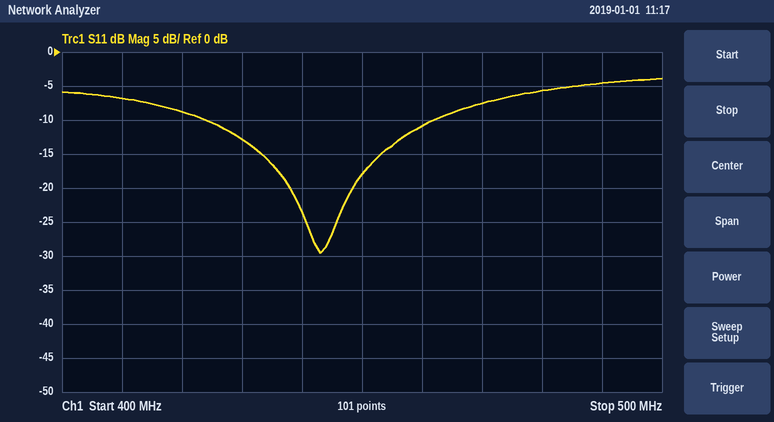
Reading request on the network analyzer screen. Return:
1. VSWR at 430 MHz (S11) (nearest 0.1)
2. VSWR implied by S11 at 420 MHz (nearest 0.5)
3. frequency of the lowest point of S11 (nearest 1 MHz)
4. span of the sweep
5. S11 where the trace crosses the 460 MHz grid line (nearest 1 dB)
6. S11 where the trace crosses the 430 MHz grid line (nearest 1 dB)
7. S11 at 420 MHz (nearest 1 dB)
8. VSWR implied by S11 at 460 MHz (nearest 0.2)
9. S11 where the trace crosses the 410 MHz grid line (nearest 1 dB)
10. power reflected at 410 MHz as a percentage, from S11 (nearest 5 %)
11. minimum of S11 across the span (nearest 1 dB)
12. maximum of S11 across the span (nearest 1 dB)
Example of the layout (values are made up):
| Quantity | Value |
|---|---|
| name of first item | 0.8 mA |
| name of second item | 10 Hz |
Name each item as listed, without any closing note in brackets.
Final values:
| Quantity | Value |
|---|---|
| VSWR at 430 MHz (S11) | 1.6 |
| VSWR implied by S11 at 420 MHz | 2.0 |
| frequency of the lowest point of S11 | 443 MHz |
| span of the sweep | 100 MHz |
| S11 where the trace crosses the 460 MHz grid line | -11 dB |
| S11 where the trace crosses the 430 MHz grid line | -13 dB |
| S11 at 420 MHz | -9 dB |
| VSWR implied by S11 at 460 MHz | 1.8 |
| S11 where the trace crosses the 410 MHz grid line | -7 dB |
| power reflected at 410 MHz as a percentage, from S11 | 20 % |
| minimum of S11 across the span | -30 dB |
| maximum of S11 across the span | -4 dB |
